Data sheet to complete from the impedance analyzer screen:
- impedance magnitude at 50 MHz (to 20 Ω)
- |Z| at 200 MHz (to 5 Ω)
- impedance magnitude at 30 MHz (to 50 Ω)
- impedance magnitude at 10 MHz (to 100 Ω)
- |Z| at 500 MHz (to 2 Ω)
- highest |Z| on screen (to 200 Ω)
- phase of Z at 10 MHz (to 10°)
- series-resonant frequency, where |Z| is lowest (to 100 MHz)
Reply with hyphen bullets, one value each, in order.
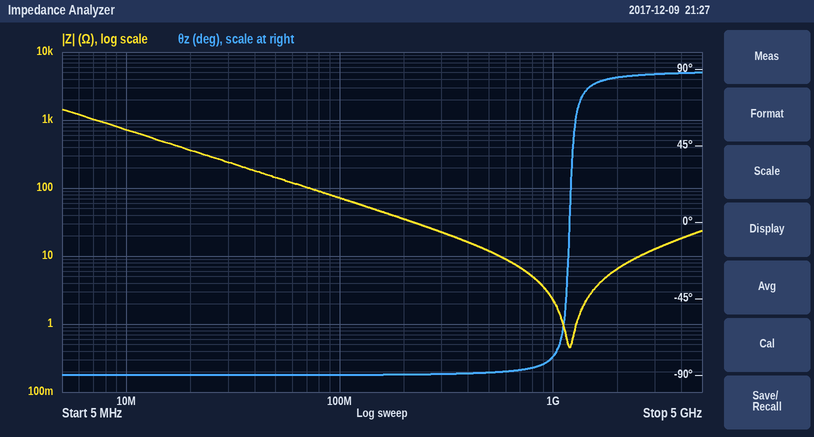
- 140 Ω
- 35 Ω
- 250 Ω
- 700 Ω
- 12 Ω
- 1.4 kΩ
- -90°
- 1.2 GHz
